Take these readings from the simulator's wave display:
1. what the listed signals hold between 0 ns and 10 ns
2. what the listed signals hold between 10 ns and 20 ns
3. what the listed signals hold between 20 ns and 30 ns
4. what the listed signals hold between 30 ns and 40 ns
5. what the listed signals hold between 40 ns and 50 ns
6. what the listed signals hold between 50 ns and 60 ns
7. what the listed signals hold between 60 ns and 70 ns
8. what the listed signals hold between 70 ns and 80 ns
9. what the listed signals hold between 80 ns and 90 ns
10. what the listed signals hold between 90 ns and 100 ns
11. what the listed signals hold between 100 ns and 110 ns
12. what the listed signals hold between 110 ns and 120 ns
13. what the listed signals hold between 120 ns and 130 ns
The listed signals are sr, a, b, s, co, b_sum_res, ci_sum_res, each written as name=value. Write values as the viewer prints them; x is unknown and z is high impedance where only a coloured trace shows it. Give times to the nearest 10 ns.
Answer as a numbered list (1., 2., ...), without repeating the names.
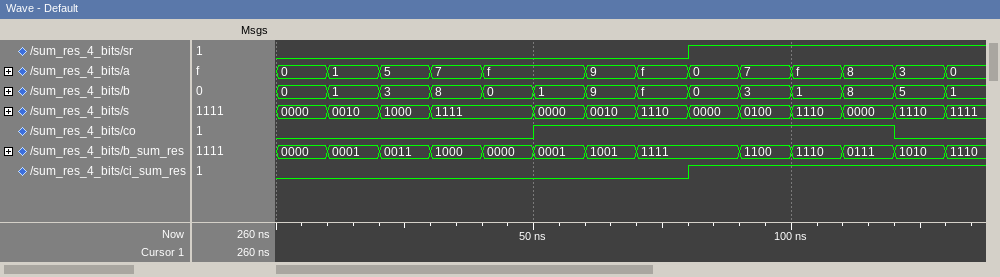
1. sr=0, a=0, b=0, s=0000, co=0, b_sum_res=0000, ci_sum_res=0
2. sr=0, a=1, b=1, s=0010, co=0, b_sum_res=0001, ci_sum_res=0
3. sr=0, a=5, b=3, s=1000, co=0, b_sum_res=0011, ci_sum_res=0
4. sr=0, a=7, b=8, s=1111, co=0, b_sum_res=1000, ci_sum_res=0
5. sr=0, a=f, b=0, s=1111, co=0, b_sum_res=0000, ci_sum_res=0
6. sr=0, a=f, b=1, s=0000, co=1, b_sum_res=0001, ci_sum_res=0
7. sr=0, a=9, b=9, s=0010, co=1, b_sum_res=1001, ci_sum_res=0
8. sr=0, a=f, b=f, s=1110, co=1, b_sum_res=1111, ci_sum_res=0
9. sr=1, a=0, b=0, s=0000, co=1, b_sum_res=1111, ci_sum_res=1
10. sr=1, a=7, b=3, s=0100, co=1, b_sum_res=1100, ci_sum_res=1
11. sr=1, a=f, b=1, s=1110, co=1, b_sum_res=1110, ci_sum_res=1
12. sr=1, a=8, b=8, s=0000, co=1, b_sum_res=0111, ci_sum_res=1
13. sr=1, a=3, b=5, s=1110, co=0, b_sum_res=1010, ci_sum_res=1
